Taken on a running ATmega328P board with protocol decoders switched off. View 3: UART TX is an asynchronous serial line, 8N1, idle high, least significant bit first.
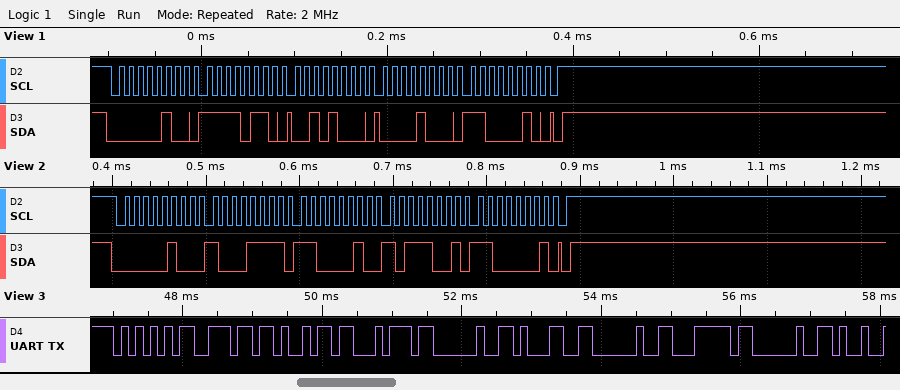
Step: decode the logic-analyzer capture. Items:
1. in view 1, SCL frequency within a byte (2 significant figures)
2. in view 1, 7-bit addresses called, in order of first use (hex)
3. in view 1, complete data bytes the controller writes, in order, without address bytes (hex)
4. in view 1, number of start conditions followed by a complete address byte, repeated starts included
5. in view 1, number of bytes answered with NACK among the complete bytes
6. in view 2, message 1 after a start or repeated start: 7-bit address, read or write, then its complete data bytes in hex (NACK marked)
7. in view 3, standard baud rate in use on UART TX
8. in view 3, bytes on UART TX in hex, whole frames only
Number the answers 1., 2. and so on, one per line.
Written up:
1. 100 kHz
2. 0x02
3. F6 28 08 C2
4. 1
5. 0
6. 0x02 write: 8F C2 B9 C1
7. 9600 baud
8. 55 6E 69 74 20 31 20 7C 20
